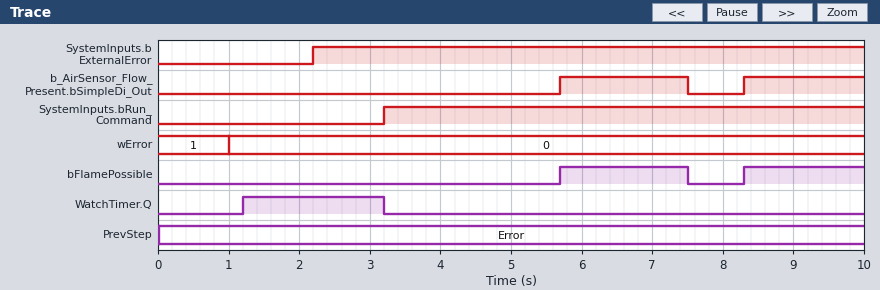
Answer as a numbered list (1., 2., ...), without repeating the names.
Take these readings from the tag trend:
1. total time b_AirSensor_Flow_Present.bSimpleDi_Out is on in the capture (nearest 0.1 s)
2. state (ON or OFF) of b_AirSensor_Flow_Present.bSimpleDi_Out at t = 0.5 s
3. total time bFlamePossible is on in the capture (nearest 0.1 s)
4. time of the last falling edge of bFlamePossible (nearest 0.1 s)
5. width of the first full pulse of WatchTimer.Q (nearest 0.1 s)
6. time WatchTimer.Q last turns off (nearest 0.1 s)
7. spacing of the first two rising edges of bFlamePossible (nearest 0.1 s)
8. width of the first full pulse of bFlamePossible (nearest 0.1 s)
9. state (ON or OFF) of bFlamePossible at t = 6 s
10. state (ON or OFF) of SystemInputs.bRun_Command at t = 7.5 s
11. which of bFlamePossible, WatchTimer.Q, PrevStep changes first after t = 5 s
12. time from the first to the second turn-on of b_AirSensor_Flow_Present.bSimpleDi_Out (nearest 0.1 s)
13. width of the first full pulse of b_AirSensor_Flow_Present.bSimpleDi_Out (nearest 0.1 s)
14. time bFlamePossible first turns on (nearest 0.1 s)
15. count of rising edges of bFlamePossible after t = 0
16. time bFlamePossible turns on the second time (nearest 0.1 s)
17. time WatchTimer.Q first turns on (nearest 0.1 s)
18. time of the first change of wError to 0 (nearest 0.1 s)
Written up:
1. 3.5 s
2. OFF
3. 3.5 s
4. 7.5 s
5. 2.0 s
6. 3.2 s
7. 2.6 s
8. 1.8 s
9. ON
10. ON
11. bFlamePossible
12. 2.6 s
13. 1.8 s
14. 5.7 s
15. 2
16. 8.3 s
17. 1.2 s
18. 1.0 s
